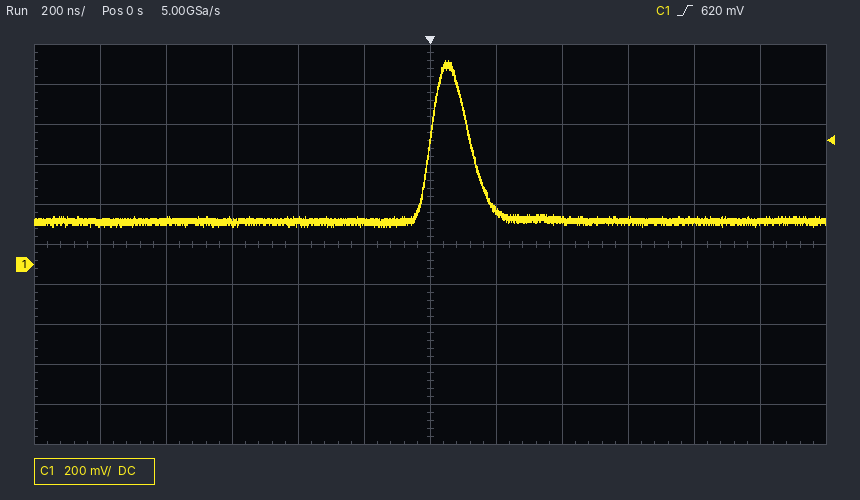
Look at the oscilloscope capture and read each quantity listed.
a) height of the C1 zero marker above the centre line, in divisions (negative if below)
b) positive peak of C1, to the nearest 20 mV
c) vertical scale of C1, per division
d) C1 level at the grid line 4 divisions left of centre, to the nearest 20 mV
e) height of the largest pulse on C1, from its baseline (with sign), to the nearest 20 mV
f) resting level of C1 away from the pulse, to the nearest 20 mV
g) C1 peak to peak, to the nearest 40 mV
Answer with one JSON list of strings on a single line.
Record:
["-0.5 div", "1.02 V", "200 mV", "220 mV", "+800 mV", "220 mV", "840 mV"]
